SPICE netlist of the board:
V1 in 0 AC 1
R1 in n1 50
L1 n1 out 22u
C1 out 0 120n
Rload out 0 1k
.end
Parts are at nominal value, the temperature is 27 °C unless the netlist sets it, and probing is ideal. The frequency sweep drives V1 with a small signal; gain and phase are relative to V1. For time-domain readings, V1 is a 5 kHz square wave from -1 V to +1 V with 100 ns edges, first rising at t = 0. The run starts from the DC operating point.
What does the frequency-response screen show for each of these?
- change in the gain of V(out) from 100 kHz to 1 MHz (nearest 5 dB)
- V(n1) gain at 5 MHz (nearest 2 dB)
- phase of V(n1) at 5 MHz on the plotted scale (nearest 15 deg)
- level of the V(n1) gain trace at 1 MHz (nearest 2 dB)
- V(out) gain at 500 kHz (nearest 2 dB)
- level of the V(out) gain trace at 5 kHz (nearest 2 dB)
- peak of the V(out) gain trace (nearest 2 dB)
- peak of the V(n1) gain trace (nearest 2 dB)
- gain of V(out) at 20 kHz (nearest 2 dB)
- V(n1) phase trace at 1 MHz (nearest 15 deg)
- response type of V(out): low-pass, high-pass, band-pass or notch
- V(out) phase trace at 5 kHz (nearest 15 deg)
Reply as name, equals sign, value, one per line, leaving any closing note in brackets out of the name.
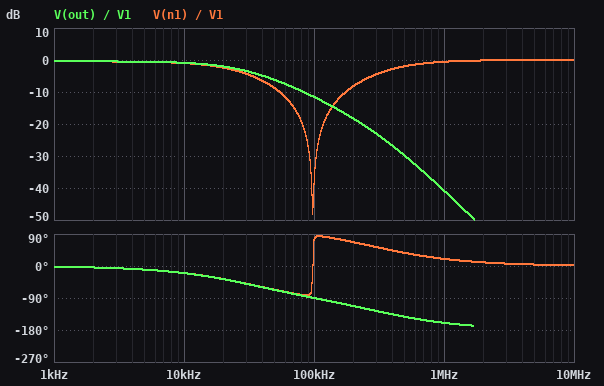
change in the gain of V(out) from 100 kHz to 1 MHz = -30 dB
V(n1) gain at 5 MHz = 0 dB
phase of V(n1) at 5 MHz on the plotted scale = 0 deg
level of the V(n1) gain trace at 1 MHz = 0 dB
V(out) gain at 500 kHz = -30 dB
level of the V(out) gain trace at 5 kHz = 0 dB
peak of the V(out) gain trace = 0 dB
peak of the V(n1) gain trace = 0 dB
gain of V(out) at 20 kHz = -2 dB
V(n1) phase trace at 1 MHz = 15 deg
response type of V(out): low-pass, high-pass, band-pass or notch = low-pass
V(out) phase trace at 5 kHz = -15 deg
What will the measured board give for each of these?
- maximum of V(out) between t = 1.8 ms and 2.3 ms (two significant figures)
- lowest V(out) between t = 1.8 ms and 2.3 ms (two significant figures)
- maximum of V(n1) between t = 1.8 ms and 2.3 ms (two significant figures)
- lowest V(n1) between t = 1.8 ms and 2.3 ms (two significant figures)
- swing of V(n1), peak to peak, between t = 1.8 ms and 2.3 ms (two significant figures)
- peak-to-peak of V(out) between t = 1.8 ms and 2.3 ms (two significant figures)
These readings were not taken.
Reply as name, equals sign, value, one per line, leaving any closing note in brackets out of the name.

maximum of V(out) between t = 1.8 ms and 2.3 ms = 950 mV
lowest V(out) between t = 1.8 ms and 2.3 ms = -950 mV
maximum of V(n1) between t = 1.8 ms and 2.3 ms = 950 mV
lowest V(n1) between t = 1.8 ms and 2.3 ms = -950 mV
swing of V(n1), peak to peak, between t = 1.8 ms and 2.3 ms = 1.9 V
peak-to-peak of V(out) between t = 1.8 ms and 2.3 ms = 1.9 V
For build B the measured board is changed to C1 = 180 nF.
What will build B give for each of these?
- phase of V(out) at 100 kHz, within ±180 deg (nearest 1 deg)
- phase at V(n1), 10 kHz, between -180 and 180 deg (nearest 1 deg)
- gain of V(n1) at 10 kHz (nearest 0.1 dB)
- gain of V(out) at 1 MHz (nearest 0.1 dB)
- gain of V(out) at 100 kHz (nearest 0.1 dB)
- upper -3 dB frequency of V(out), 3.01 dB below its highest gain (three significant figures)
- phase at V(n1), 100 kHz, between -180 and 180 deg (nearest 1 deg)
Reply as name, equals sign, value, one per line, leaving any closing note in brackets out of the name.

phase of V(out) at 100 kHz, within ±180 deg = -95 deg
phase at V(n1), 10 kHz, between -180 and 180 deg = -29 deg
gain of V(n1) at 10 kHz = -1.6 dB
gain of V(out) at 1 MHz = -44.4 dB
gain of V(out) at 100 kHz = -15.1 dB
upper -3 dB frequency of V(out), 3.01 dB below its highest gain = 19.5 kHz
phase at V(n1), 100 kHz, between -180 and 180 deg = 83 deg
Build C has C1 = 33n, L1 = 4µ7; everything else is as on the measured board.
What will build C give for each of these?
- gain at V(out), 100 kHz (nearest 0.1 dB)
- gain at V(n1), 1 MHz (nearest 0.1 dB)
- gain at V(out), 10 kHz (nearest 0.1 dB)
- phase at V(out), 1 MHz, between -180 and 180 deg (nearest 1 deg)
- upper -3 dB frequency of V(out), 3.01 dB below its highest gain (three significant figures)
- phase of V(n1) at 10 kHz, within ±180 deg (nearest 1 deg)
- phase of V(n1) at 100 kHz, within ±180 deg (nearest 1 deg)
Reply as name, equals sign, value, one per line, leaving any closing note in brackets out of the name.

gain at V(out), 100 kHz = -3.1 dB
gain at V(n1), 1 MHz = -7.1 dB
gain at V(out), 10 kHz = -0.5 dB
phase at V(out), 1 MHz, between -180 and 180 deg = -116 deg
upper -3 dB frequency of V(out), 3.01 dB below its highest gain = 107 kHz
phase of V(n1) at 10 kHz, within ±180 deg = -6 deg
phase of V(n1) at 100 kHz, within ±180 deg = -46 deg
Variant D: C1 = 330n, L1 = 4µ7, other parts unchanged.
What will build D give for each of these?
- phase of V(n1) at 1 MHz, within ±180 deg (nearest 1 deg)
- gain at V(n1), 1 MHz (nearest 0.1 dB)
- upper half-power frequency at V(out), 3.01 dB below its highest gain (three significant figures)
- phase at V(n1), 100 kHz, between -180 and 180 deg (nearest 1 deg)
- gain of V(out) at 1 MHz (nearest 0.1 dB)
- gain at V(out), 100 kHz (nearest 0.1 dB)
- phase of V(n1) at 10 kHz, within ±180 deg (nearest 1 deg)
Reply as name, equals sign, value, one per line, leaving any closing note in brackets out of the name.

phase of V(n1) at 1 MHz, within ±180 deg = 60 deg
gain at V(n1), 1 MHz = -6.0 dB
upper half-power frequency at V(out), 3.01 dB below its highest gain = 10.2 kHz
phase at V(n1), 100 kHz, between -180 and 180 deg = -87 deg
gain of V(out) at 1 MHz = -41.6 dB
gain at V(out), 100 kHz = -20.3 dB
phase of V(n1) at 10 kHz, within ±180 deg = -45 deg
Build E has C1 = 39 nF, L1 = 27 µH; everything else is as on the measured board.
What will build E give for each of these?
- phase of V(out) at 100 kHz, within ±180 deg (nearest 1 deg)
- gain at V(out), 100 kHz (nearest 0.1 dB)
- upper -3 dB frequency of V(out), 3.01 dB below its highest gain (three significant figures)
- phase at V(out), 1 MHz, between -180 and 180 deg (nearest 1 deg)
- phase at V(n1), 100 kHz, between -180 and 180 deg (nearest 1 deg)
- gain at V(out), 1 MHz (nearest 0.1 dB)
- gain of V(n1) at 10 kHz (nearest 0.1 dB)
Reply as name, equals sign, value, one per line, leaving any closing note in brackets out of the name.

phase of V(out) at 100 kHz, within ±180 deg = -63 deg
gain at V(out), 100 kHz = -2.9 dB
upper -3 dB frequency of V(out), 3.01 dB below its highest gain = 112 kHz
phase at V(out), 1 MHz, between -180 and 180 deg = -163 deg
phase at V(n1), 100 kHz, between -180 and 180 deg = -61 deg
gain at V(out), 1 MHz = -32.5 dB
gain of V(n1) at 10 kHz = -0.5 dB
